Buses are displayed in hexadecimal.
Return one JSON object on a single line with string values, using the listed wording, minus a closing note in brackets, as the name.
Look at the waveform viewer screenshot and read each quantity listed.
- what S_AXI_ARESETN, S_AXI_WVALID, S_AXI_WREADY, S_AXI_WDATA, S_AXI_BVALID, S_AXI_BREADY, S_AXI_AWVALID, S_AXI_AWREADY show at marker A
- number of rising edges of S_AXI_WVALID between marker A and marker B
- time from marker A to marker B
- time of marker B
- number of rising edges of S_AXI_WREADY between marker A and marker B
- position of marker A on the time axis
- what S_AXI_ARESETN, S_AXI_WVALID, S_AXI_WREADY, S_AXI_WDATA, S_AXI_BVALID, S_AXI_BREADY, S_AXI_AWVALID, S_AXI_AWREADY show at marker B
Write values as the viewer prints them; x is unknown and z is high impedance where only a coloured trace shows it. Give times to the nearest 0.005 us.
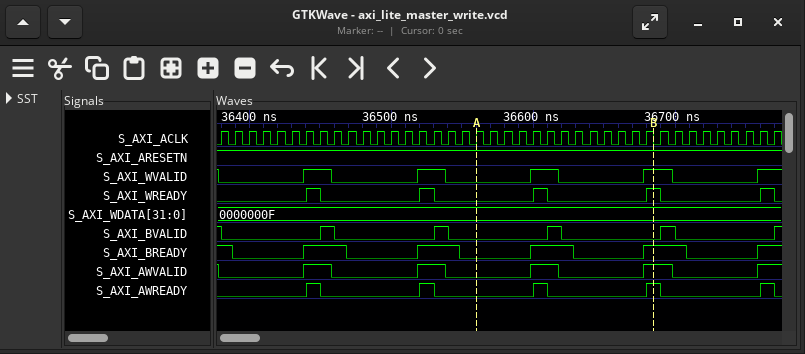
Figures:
{"what S_AXI_ARESETN, S_AXI_WVALID, S_AXI_WREADY, S_AXI_WDATA, S_AXI_BVALID, S_AXI_BREADY, S_AXI_AWVALID, S_AXI_AWREADY show at marker A": "S_AXI_ARESETN=1, S_AXI_WVALID=0, S_AXI_WREADY=0, S_AXI_WDATA=0000000F, S_AXI_BVALID=0, S_AXI_BREADY=0, S_AXI_AWVALID=0, S_AXI_AWREADY=0", "number of rising edges of S_AXI_WVALID between marker A and marker B": "2", "time from marker A to marker B": "0.125 us", "time of marker B": "36.685 us", "number of rising edges of S_AXI_WREADY between marker A and marker B": "2", "position of marker A on the time axis": "36.56 us", "what S_AXI_ARESETN, S_AXI_WVALID, S_AXI_WREADY, S_AXI_WDATA, S_AXI_BVALID, S_AXI_BREADY, S_AXI_AWVALID, S_AXI_AWREADY show at marker B": "S_AXI_ARESETN=1, S_AXI_WVALID=1, S_AXI_WREADY=1, S_AXI_WDATA=0000000F, S_AXI_BVALID=0, S_AXI_BREADY=1, S_AXI_AWVALID=1, S_AXI_AWREADY=1"}
